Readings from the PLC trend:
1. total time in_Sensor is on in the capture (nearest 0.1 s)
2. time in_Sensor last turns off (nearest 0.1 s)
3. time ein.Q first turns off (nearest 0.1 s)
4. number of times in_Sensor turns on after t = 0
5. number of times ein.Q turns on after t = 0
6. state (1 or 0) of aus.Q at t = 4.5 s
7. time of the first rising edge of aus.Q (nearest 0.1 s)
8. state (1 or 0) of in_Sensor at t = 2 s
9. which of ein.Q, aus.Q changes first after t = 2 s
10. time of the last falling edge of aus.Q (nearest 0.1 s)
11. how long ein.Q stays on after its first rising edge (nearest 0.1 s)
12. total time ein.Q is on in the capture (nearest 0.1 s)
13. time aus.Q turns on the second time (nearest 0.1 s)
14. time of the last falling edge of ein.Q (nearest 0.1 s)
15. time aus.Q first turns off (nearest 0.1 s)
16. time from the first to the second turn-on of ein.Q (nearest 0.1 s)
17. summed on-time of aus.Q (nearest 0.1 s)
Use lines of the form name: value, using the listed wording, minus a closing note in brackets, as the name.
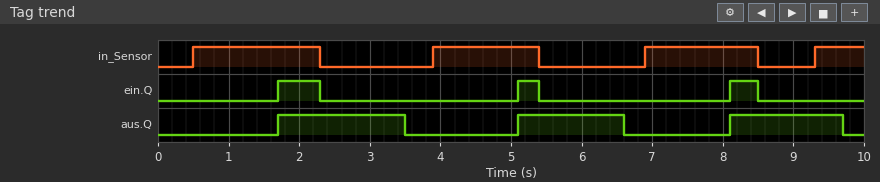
total time in_Sensor is on in the capture: 5.6 s
time in_Sensor last turns off: 8.5 s
time ein.Q first turns off: 2.3 s
number of times in_Sensor turns on after t = 0: 4
number of times ein.Q turns on after t = 0: 3
state (1 or 0) of aus.Q at t = 4.5 s: 0
time of the first rising edge of aus.Q: 1.7 s
state (1 or 0) of in_Sensor at t = 2 s: 1
which of ein.Q, aus.Q changes first after t = 2 s: ein.Q
time of the last falling edge of aus.Q: 9.7 s
how long ein.Q stays on after its first rising edge: 0.6 s
total time ein.Q is on in the capture: 1.3 s
time aus.Q turns on the second time: 5.1 s
time of the last falling edge of ein.Q: 8.5 s
time aus.Q first turns off: 3.5 s
time from the first to the second turn-on of ein.Q: 3.4 s
summed on-time of aus.Q: 4.9 s
